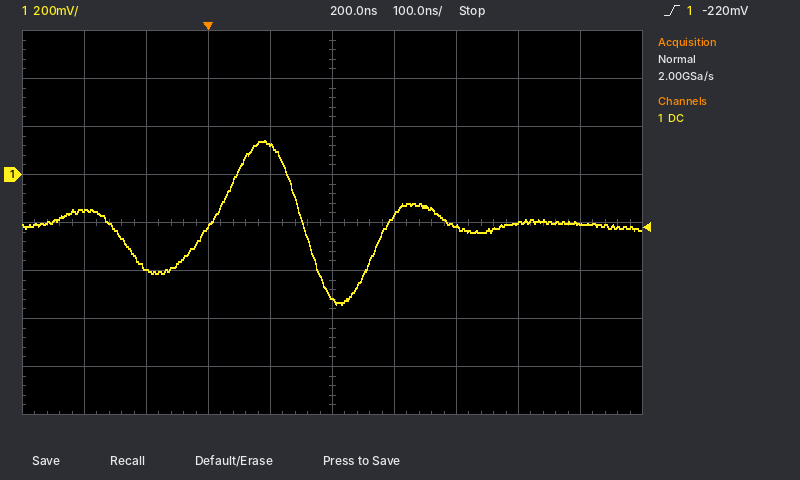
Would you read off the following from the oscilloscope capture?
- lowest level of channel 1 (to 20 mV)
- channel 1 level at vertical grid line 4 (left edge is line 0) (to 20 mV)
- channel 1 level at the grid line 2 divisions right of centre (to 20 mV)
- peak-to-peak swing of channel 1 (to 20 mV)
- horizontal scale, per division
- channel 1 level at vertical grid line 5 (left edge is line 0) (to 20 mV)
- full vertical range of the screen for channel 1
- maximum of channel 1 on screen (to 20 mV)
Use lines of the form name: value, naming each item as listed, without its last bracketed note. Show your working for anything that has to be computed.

lowest level of channel 1: -540 mV
channel 1 level at vertical grid line 4 (left edge is line 0): 120 mV
channel 1 level at the grid line 2 divisions right of centre: -220 mV
peak-to-peak swing of channel 1: 140 mV − (-540 mV) = 680 mV
horizontal scale, per division: 100 ns
channel 1 level at vertical grid line 5 (left edge is line 0): -520 mV
full vertical range of the screen for channel 1: 1.6 V
maximum of channel 1 on screen: 140 mV
